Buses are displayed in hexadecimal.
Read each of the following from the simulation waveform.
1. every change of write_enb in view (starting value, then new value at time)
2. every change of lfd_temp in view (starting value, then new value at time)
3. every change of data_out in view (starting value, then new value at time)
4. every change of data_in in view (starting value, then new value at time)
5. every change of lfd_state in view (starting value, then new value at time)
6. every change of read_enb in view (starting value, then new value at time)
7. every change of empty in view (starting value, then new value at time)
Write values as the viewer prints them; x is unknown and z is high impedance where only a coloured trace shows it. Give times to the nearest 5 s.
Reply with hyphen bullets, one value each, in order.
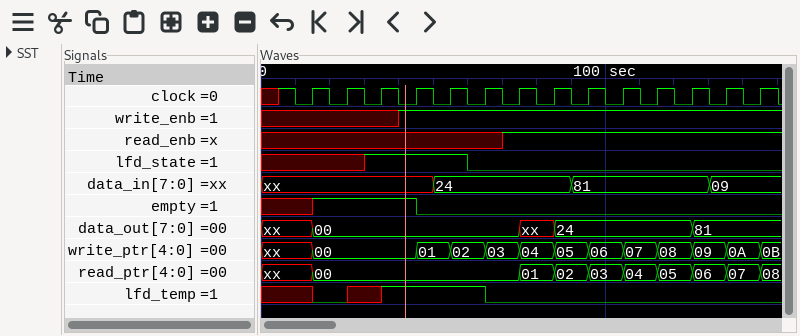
- x, 1 at 40 s
- x, 0 at 15 s, x at 25 s, 1 at 35 s, 0 at 65 s
- xx, 00 at 15 s, xx at 75 s, 24 at 85 s, 81 at 125 s
- xx, 24 at 50 s, 81 at 90 s, 09 at 130 s
- x, 1 at 30 s, 0 at 60 s
- x, 1 at 70 s
- x, 1 at 15 s, 0 at 45 s
